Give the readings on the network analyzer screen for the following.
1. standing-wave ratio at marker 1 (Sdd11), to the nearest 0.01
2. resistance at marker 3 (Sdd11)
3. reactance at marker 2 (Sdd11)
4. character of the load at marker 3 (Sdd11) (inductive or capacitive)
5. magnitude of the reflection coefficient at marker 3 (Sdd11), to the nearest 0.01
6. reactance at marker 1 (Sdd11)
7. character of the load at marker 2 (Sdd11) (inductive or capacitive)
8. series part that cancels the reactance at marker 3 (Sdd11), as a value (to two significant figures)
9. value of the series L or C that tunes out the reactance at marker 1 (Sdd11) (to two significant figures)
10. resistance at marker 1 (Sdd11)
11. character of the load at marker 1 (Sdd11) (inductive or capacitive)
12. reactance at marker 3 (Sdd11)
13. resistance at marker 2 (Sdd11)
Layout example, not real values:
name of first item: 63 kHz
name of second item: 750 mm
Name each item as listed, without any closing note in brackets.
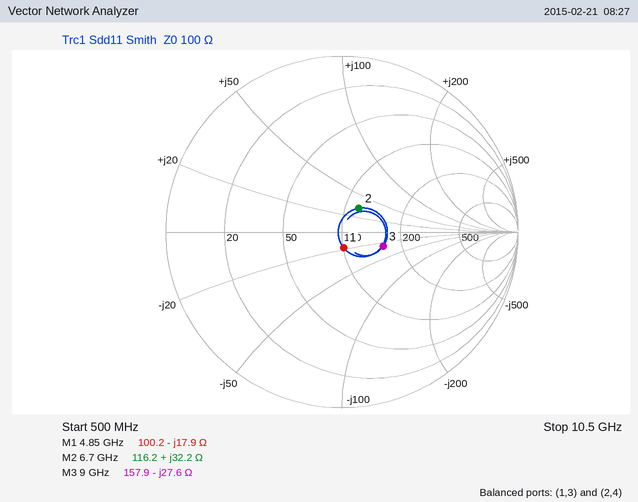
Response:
standing-wave ratio at marker 1 (Sdd11), to the nearest 0.01: 1.20
resistance at marker 3: 157.9 Ω
reactance at marker 2: +32.2 Ω
character of the load at marker 3 (Sdd11): capacitive
magnitude of the reflection coefficient at marker 3 (Sdd11), to the nearest 0.01: 0.25
reactance at marker 1: -17.9 Ω
character of the load at marker 2 (Sdd11): inductive
series part that cancels the reactance at marker 3 (Sdd11), as a value: 490 pH
value of the series L or C that tunes out the reactance at marker 1 (Sdd11): 590 pH
resistance at marker 1: 100.2 Ω
character of the load at marker 1 (Sdd11): capacitive
reactance at marker 3: -27.6 Ω
resistance at marker 2: 116.2 Ω
